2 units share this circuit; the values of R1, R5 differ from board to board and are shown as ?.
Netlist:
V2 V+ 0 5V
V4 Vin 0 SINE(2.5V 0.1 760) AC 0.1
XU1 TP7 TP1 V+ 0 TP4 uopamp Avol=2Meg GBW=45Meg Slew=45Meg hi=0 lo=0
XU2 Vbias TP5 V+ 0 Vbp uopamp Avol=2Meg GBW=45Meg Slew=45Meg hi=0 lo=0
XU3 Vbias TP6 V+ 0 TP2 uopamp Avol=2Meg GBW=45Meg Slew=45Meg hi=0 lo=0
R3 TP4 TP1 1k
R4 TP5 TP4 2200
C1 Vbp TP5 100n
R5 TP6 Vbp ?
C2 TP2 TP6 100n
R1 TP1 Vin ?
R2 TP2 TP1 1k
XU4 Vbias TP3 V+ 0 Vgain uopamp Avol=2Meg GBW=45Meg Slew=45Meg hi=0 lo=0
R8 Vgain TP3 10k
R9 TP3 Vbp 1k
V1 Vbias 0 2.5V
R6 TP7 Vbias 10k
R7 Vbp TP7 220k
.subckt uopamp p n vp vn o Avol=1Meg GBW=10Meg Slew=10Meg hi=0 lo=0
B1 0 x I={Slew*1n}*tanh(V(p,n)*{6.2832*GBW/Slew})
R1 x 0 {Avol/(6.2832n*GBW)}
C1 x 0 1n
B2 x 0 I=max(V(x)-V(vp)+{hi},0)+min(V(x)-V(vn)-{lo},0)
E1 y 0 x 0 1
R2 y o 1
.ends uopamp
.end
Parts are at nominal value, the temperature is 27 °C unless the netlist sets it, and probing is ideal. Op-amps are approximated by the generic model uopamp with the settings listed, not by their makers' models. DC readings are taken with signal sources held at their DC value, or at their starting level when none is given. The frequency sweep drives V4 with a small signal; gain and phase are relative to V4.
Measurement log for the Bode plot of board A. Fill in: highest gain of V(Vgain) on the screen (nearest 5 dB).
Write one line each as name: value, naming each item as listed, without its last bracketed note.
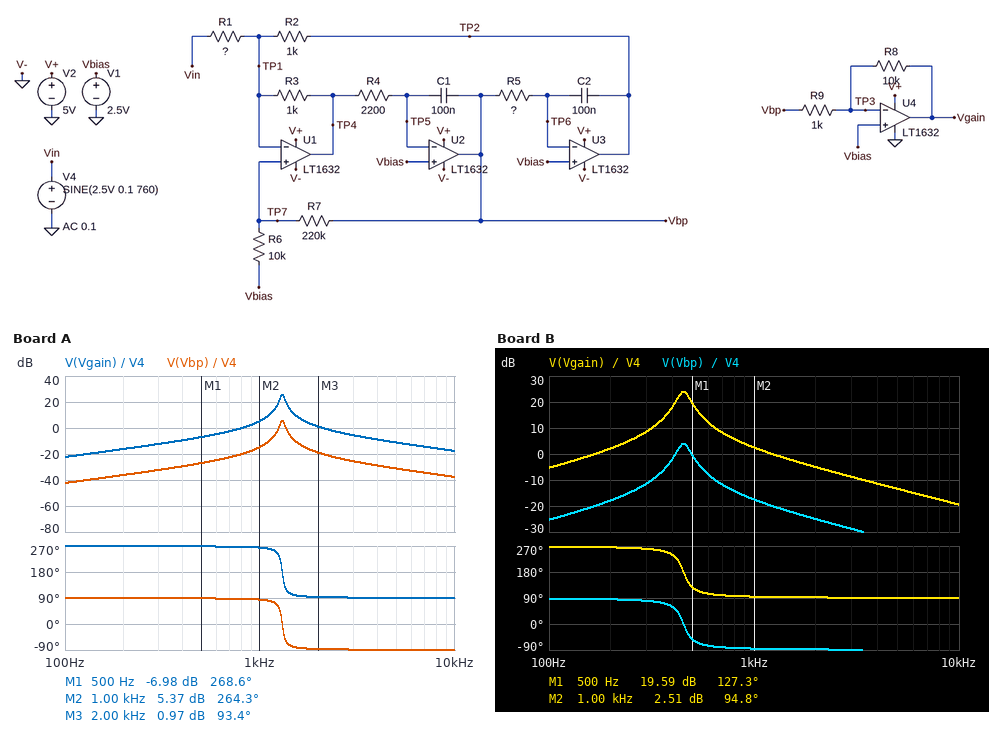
highest gain of V(Vgain) on the screen: 25 dB
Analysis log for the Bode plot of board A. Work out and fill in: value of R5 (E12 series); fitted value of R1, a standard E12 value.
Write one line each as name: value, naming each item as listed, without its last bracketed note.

value of R5: 680 Ω
fitted value of R1, a standard E12 value: 5.6 kΩ
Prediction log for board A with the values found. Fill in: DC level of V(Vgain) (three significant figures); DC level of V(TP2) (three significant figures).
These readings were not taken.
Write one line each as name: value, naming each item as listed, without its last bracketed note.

DC level of V(Vgain): 2.50 V
DC level of V(TP2): 2.50 V
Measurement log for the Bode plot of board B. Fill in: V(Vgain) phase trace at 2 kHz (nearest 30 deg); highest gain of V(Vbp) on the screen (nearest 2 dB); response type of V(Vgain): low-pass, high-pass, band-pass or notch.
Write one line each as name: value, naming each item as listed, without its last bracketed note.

V(Vgain) phase trace at 2 kHz: 90 deg
highest gain of V(Vbp) on the screen: 4 dB
response type of V(Vgain): low-pass, high-pass, band-pass or notch: band-pass
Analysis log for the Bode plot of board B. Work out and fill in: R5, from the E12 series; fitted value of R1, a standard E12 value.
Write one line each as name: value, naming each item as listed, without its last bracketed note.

R5, from the E12 series: 5.6 kΩ
fitted value of R1, a standard E12 value: 6.8 kΩ
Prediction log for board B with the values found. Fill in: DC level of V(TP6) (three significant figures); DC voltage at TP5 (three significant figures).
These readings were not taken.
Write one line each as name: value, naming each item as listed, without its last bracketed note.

DC level of V(TP6): 2.50 V
DC voltage at TP5: 2.50 V
